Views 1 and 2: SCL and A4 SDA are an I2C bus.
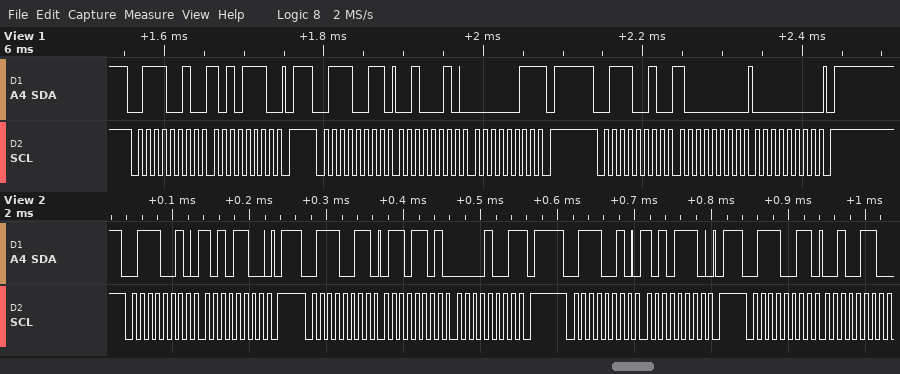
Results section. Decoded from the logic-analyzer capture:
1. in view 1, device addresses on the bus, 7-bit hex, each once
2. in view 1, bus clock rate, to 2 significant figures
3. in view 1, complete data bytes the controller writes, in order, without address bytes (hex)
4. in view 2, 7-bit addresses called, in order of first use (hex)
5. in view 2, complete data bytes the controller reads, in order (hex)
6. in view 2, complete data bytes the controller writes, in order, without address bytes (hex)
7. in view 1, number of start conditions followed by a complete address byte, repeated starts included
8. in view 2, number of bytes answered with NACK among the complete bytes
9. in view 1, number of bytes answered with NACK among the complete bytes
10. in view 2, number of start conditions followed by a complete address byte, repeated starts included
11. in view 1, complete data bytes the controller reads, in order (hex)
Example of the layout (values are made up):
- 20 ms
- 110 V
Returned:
- 0x39
- 100 kHz
- AE 80 00
- 0x39
- 6D 09 26
- AC AE
- 3
- 1
- 1
- 4
- 22 03
